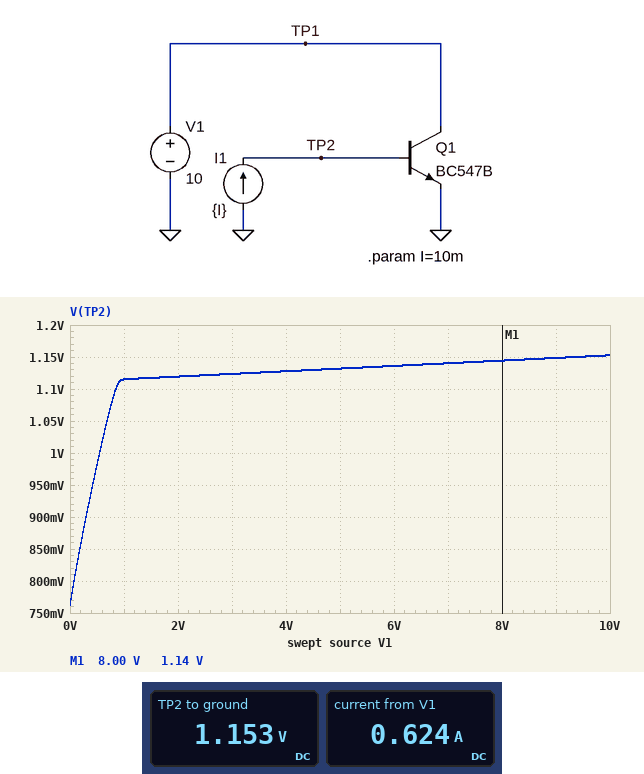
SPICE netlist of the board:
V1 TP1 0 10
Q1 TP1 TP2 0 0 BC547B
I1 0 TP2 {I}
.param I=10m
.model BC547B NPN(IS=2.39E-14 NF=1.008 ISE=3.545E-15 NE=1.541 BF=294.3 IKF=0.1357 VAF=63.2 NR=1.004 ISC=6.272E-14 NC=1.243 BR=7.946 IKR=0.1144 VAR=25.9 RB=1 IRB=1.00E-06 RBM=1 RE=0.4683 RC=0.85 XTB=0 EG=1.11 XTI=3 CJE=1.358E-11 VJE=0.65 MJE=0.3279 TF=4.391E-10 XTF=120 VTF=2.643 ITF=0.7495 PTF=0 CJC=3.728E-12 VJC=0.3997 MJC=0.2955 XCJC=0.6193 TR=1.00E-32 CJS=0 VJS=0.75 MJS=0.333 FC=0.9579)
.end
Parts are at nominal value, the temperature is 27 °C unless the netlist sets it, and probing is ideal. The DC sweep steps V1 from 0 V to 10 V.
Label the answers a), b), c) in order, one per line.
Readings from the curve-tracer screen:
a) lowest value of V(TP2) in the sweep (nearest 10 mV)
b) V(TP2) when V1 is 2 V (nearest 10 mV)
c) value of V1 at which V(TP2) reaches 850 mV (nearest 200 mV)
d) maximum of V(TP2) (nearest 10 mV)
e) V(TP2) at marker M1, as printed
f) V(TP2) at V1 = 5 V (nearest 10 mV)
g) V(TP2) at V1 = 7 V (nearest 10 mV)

a) 760 mV
b) 1.12 V
c) 200 mV
d) 1.15 V
e) 1.14 V
f) 1.13 V
g) 1.14 V
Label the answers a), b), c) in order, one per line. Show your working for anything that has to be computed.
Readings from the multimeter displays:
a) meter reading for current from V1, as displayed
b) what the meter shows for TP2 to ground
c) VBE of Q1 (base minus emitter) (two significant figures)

a) 0.624 A
b) 1.153 V
c) 1.153 V = 1.2 V
